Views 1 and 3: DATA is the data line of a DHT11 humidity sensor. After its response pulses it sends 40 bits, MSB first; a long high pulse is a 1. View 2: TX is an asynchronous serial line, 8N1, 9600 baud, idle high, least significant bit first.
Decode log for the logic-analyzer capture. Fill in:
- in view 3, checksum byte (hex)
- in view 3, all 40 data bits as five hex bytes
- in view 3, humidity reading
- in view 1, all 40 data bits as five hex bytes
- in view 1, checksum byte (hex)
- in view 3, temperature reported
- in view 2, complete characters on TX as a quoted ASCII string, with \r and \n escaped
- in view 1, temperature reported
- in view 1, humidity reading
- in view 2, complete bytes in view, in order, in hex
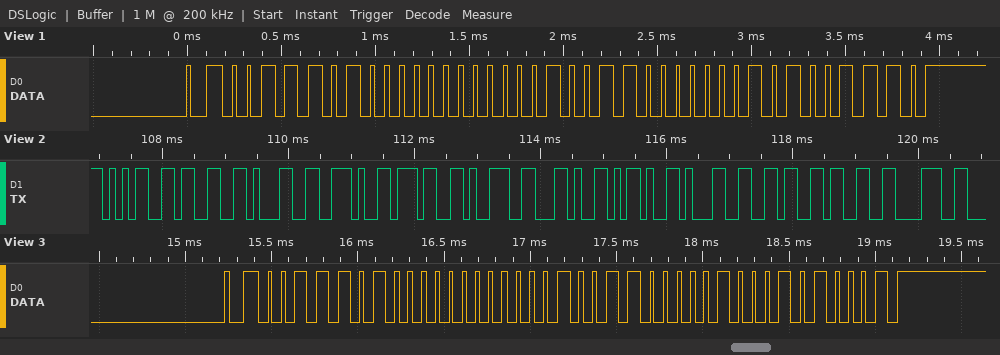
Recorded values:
0x51
3A 00 13 04 51
58 %
3A 00 13 01 4E
0x4E
19.4 °C
"531.79,-1638"
19.1 °C
58 %
35 33 31 2E 37 39 2C 2D 31 36 33 38
